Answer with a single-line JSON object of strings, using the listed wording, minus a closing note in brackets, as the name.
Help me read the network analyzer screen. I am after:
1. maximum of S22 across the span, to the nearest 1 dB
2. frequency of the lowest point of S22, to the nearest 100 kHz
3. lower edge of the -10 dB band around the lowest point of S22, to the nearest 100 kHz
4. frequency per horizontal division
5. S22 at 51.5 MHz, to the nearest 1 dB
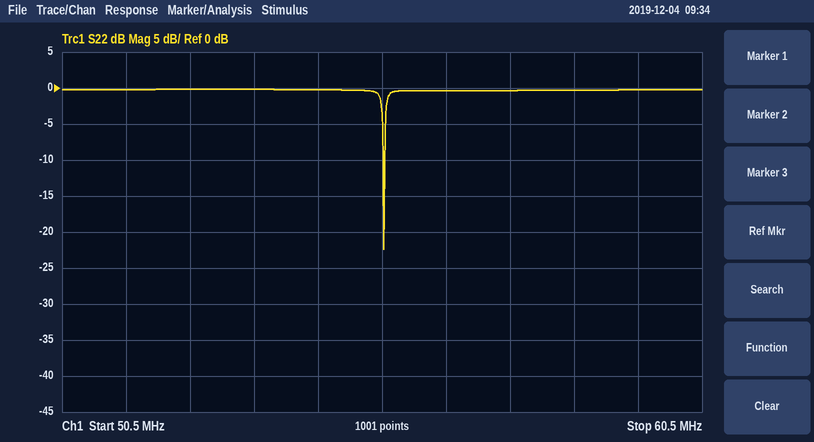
{"maximum of S22 across the span, to the nearest 1 dB": "0 dB", "frequency of the lowest point of S22, to the nearest 100 kHz": "55.5 MHz", "lower edge of the -10 dB band around the lowest point of S22, to the nearest 100 kHz": "55.5 MHz", "frequency per horizontal division": "1 MHz", "S22 at 51.5 MHz, to the nearest 1 dB": "0 dB"}
